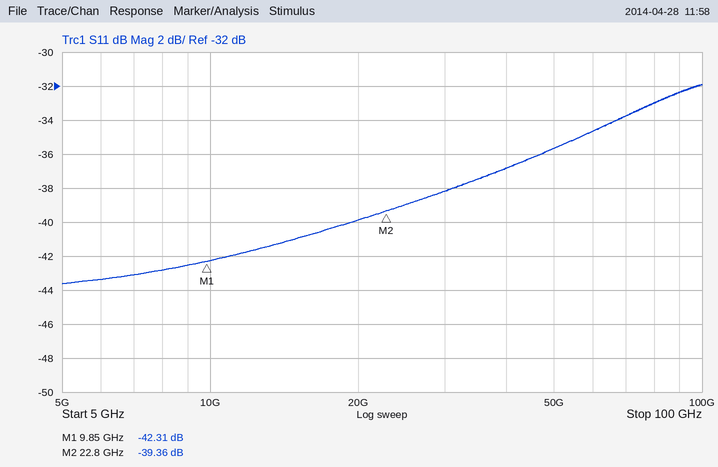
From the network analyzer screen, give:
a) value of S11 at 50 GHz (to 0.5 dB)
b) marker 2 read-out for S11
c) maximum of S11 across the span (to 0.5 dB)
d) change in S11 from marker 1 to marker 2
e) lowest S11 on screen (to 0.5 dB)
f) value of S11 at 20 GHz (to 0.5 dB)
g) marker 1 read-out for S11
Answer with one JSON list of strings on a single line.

["-35.5 dB", "-39.36 dB", "-32.0 dB", "2.95 dB", "-43.5 dB", "-40.0 dB", "-42.31 dB"]
